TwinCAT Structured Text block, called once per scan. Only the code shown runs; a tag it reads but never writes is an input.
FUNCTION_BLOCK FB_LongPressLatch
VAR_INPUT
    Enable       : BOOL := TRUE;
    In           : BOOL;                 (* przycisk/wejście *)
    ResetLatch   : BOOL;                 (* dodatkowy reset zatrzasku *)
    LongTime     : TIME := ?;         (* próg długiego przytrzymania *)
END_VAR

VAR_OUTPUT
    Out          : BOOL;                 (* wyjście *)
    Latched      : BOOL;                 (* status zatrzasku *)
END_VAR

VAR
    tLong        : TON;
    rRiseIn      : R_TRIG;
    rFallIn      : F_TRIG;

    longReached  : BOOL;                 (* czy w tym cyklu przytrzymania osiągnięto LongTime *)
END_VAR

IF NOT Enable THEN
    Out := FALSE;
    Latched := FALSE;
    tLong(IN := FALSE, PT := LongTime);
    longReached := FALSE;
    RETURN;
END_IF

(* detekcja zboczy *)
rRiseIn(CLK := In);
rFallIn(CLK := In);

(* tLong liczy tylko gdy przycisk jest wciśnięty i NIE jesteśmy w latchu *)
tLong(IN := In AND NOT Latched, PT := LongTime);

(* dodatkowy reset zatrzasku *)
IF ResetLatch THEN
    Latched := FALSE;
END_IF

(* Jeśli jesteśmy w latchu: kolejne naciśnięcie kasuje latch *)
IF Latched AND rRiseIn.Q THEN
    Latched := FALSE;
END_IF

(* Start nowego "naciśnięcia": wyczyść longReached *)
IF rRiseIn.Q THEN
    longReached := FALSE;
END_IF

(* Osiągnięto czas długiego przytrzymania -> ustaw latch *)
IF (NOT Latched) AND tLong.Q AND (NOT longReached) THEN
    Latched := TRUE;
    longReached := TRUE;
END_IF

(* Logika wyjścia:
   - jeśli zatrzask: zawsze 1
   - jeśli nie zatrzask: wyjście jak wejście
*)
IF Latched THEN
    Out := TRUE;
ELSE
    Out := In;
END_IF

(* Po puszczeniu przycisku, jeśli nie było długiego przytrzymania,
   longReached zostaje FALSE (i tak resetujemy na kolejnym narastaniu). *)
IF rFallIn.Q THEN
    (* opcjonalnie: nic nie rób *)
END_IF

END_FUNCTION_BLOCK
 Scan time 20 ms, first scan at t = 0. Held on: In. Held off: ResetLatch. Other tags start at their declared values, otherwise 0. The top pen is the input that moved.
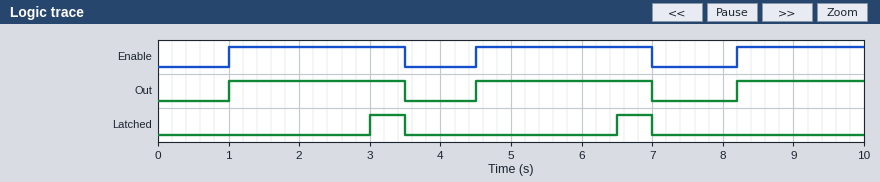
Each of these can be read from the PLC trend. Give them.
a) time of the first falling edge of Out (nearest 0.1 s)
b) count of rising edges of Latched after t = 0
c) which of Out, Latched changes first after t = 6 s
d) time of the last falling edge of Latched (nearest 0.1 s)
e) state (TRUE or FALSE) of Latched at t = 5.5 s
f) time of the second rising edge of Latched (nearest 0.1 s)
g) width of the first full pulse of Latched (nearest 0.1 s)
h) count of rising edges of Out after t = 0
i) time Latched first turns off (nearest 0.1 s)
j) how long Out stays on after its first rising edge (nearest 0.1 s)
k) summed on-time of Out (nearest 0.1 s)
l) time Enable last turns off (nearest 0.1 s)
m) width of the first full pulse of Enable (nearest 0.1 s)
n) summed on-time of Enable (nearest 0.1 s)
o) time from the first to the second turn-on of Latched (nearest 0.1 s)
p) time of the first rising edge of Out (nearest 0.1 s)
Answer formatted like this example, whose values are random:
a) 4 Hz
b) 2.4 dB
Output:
a) 3.5 s
b) 2
c) Latched
d) 7.0 s
e) FALSE
f) 6.5 s
g) 0.5 s
h) 3
i) 3.5 s
j) 2.5 s
k) 6.8 s
l) 7.0 s
m) 2.5 s
n) 6.8 s
o) 3.5 s
p) 1.0 s
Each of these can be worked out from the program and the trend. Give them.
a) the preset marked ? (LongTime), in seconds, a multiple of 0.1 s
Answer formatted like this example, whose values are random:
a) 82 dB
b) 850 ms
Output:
a) 2.0 s
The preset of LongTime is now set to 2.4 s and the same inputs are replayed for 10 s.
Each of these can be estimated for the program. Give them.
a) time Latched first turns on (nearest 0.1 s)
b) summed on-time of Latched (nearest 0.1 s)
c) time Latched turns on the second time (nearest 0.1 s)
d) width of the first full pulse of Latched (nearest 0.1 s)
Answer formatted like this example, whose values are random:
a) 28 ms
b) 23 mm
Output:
a) 3.4 s
b) 0.2 s
c) 6.9 s
d) 0.1 s
